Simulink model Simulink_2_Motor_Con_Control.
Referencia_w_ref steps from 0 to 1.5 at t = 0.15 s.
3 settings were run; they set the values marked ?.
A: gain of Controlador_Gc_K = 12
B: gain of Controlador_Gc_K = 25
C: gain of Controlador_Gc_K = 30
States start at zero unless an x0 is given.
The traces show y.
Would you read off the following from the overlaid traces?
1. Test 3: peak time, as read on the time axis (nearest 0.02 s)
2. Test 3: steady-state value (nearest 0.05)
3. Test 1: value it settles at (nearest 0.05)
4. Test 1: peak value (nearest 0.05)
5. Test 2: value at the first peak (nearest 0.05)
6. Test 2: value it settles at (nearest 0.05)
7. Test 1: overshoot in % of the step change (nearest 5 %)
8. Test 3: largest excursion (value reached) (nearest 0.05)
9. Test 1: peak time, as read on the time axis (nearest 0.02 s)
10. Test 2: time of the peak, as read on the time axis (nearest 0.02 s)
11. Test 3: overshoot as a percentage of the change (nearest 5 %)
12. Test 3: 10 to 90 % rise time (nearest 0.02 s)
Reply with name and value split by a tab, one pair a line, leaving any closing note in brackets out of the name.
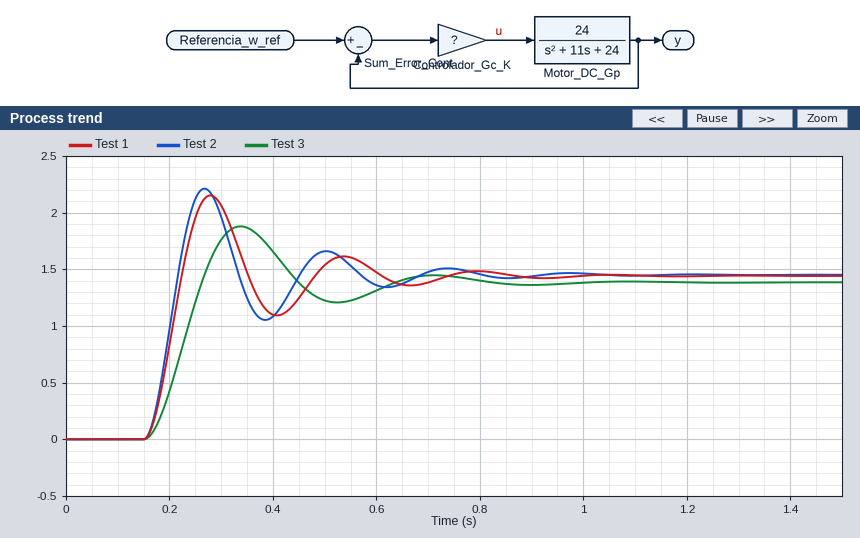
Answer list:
Test 3: peak time, as read on the time axis	0.34 s
Test 3: steady-state value	1.40
Test 1: value it settles at	1.45
Test 1: peak value	2.15
Test 2: value at the first peak	2.20
Test 2: value it settles at	1.45
Test 1: overshoot in % of the step change	50 %
Test 3: largest excursion (value reached)	1.90
Test 1: peak time, as read on the time axis	0.28 s
Test 2: time of the peak, as read on the time axis	0.26 s
Test 3: overshoot as a percentage of the change	35 %
Test 3: 10 to 90 % rise time	0.08 s
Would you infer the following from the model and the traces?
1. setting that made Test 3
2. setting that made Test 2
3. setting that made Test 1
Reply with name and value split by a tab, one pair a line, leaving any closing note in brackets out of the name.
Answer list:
setting that made Test 3	A
setting that made Test 2	C
setting that made Test 1	B
